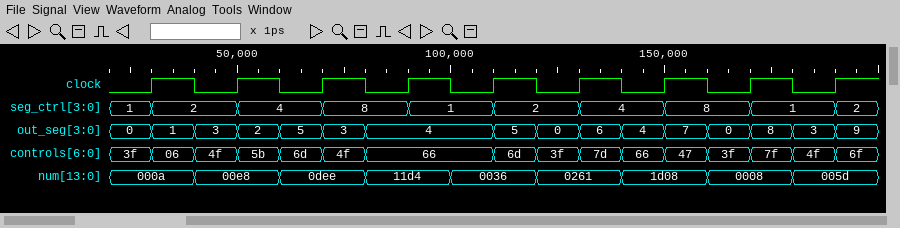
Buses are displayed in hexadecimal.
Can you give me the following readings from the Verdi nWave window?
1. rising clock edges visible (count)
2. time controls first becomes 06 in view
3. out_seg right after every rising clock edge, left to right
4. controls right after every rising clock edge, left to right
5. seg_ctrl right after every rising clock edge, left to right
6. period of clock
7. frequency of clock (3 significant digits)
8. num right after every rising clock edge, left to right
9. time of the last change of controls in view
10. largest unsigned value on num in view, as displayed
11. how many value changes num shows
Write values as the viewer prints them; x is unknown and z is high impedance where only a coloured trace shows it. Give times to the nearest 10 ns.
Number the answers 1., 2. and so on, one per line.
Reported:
1. 9
2. 30 ns
3. 1, 2, 3, 4, 5, 6, 7, 8, 9
4. 06, 5b, 4f, 66, 6d, 7d, 47, 7f, 6f
5. 2, 4, 8, 1, 2, 4, 8, 1, 2
6. 20 ns
7. 50.0 MHz
8. 000a, 00e8, 0dee, 11d4, 0036, 0261, 1d08, 0008, 005d
9. 190 ns
10. 1d08
11. 8
